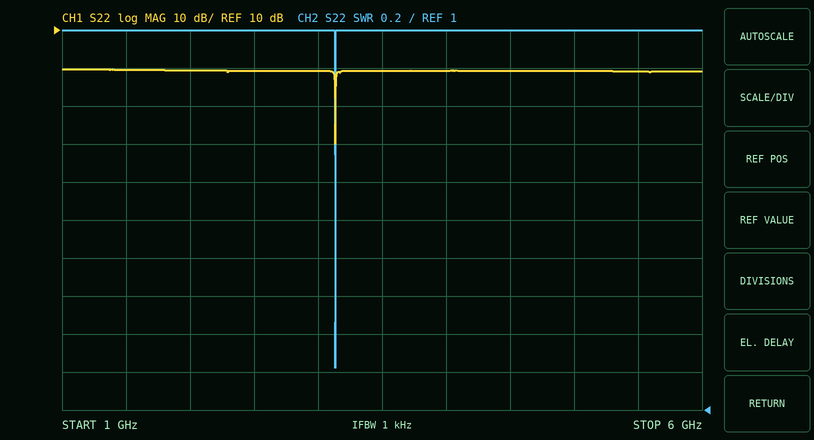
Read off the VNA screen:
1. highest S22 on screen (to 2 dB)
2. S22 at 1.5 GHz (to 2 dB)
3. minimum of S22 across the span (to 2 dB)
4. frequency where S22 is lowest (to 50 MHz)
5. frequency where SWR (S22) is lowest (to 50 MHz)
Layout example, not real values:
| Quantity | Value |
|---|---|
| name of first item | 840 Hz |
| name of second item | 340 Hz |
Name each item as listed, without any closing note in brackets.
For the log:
| Quantity | Value |
|---|---|
| highest S22 on screen | 0 dB |
| S22 at 1.5 GHz | 0 dB |
| minimum of S22 across the span | -20 dB |
| frequency where S22 is lowest | 3.15 GHz |
| frequency where SWR (S22) is lowest | 3.15 GHz |
